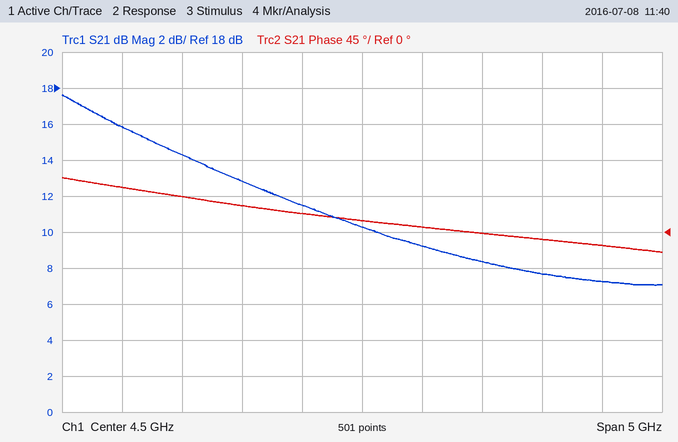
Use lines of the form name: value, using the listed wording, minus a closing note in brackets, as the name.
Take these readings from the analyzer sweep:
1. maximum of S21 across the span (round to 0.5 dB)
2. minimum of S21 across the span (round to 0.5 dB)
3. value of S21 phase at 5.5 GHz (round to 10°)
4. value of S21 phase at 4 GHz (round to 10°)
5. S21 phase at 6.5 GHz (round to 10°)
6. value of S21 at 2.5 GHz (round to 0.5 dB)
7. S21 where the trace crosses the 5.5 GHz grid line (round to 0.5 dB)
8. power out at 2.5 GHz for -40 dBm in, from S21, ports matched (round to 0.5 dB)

maximum of S21 across the span: 17.5 dB
minimum of S21 across the span: 7.0 dB
value of S21 phase at 5.5 GHz: 0°
value of S21 phase at 4 GHz: 20°
S21 phase at 6.5 GHz: -20°
value of S21 at 2.5 GHz: 16.0 dB
S21 where the trace crosses the 5.5 GHz grid line: 8.5 dB
power out at 2.5 GHz for -40 dBm in, from S21, ports matched: -24.0 dBm
